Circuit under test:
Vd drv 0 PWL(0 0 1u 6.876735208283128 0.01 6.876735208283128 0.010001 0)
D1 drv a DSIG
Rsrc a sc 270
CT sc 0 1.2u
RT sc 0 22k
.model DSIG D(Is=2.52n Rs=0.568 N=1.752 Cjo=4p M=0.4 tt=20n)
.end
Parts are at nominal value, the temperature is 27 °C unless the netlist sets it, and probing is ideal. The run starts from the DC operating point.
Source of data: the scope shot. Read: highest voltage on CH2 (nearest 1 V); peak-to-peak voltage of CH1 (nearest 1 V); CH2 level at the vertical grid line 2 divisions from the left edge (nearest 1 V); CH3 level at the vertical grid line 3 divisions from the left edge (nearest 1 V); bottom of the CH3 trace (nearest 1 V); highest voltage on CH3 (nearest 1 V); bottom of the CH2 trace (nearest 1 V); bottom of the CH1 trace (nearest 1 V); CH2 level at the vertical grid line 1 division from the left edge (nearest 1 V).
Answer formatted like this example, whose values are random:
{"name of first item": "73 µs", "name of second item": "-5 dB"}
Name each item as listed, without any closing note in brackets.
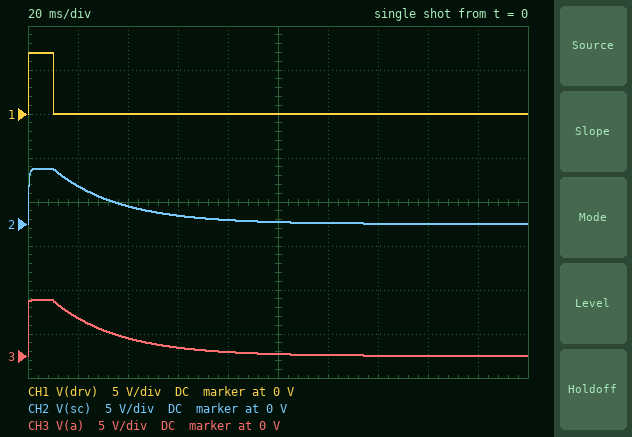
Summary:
{"highest voltage on CH2": "6 V", "peak-to-peak voltage of CH1": "7 V", "CH2 level at the vertical grid line 2 divisions from the left edge": "2 V", "CH3 level at the vertical grid line 3 divisions from the left edge": "1 V", "bottom of the CH3 trace": "0 V", "highest voltage on CH3": "6 V", "bottom of the CH2 trace": "0 V", "bottom of the CH1 trace": "0 V", "CH2 level at the vertical grid line 1 division from the left edge": "4 V"}
